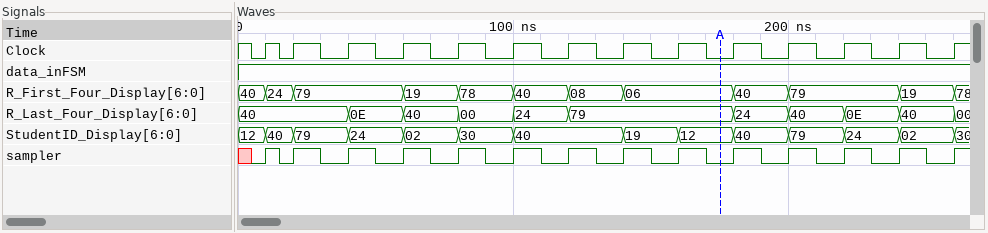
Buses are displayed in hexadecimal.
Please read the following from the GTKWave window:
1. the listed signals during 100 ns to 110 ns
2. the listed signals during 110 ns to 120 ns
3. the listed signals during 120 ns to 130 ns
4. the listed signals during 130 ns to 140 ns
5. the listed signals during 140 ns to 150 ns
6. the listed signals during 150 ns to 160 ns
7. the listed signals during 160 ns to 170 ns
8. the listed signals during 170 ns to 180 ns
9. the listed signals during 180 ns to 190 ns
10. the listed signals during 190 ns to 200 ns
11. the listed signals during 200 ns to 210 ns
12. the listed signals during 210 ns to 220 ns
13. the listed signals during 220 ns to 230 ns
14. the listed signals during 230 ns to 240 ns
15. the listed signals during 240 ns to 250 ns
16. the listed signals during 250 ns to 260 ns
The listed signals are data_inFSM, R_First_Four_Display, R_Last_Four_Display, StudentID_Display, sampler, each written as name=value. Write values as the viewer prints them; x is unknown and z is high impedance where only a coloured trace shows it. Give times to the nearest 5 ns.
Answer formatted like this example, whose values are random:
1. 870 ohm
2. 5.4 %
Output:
1. data_inFSM=1, R_First_Four_Display=40, R_Last_Four_Display=24, StudentID_Display=40, sampler=1
2. data_inFSM=1, R_First_Four_Display=40, R_Last_Four_Display=24, StudentID_Display=40, sampler=0
3. data_inFSM=1, R_First_Four_Display=08, R_Last_Four_Display=79, StudentID_Display=40, sampler=1
4. data_inFSM=1, R_First_Four_Display=08, R_Last_Four_Display=79, StudentID_Display=40, sampler=0
5. data_inFSM=1, R_First_Four_Display=06, R_Last_Four_Display=79, StudentID_Display=19, sampler=1
6. data_inFSM=1, R_First_Four_Display=06, R_Last_Four_Display=79, StudentID_Display=19, sampler=0
7. data_inFSM=1, R_First_Four_Display=06, R_Last_Four_Display=79, StudentID_Display=12, sampler=1
8. data_inFSM=1, R_First_Four_Display=06, R_Last_Four_Display=79, StudentID_Display=12, sampler=0
9. data_inFSM=1, R_First_Four_Display=40, R_Last_Four_Display=24, StudentID_Display=40, sampler=1
10. data_inFSM=1, R_First_Four_Display=40, R_Last_Four_Display=24, StudentID_Display=40, sampler=0
11. data_inFSM=1, R_First_Four_Display=79, R_Last_Four_Display=40, StudentID_Display=79, sampler=1
12. data_inFSM=1, R_First_Four_Display=79, R_Last_Four_Display=40, StudentID_Display=79, sampler=0
13. data_inFSM=1, R_First_Four_Display=79, R_Last_Four_Display=0E, StudentID_Display=24, sampler=1
14. data_inFSM=1, R_First_Four_Display=79, R_Last_Four_Display=0E, StudentID_Display=24, sampler=0
15. data_inFSM=1, R_First_Four_Display=19, R_Last_Four_Display=40, StudentID_Display=02, sampler=1
16. data_inFSM=1, R_First_Four_Display=19, R_Last_Four_Display=40, StudentID_Display=02, sampler=0
